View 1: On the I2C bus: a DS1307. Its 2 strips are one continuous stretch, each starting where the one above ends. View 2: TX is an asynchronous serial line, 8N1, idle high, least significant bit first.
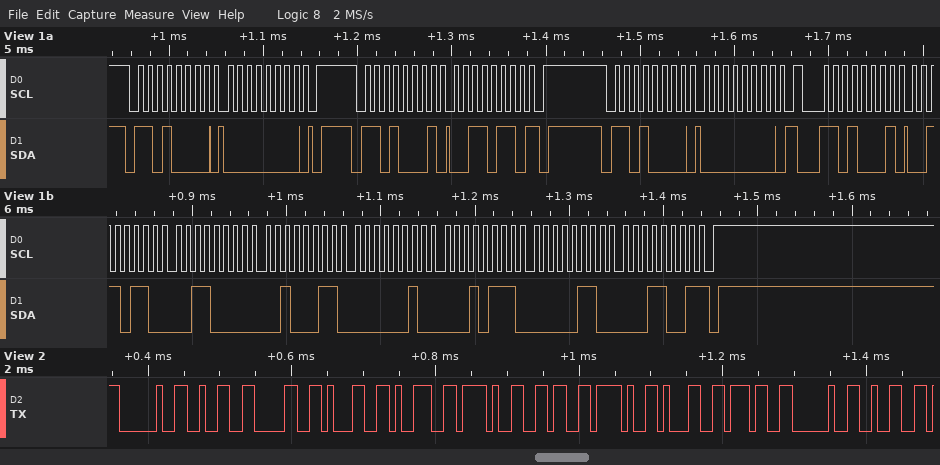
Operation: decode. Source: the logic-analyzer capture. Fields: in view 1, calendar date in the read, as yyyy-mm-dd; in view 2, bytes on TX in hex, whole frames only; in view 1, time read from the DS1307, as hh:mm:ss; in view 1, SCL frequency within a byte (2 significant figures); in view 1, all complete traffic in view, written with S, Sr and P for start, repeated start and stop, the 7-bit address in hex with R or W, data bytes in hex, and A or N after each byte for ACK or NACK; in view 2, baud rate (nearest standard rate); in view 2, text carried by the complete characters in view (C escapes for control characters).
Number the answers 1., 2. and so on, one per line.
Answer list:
1. 2019-06-17
2. 20 32 30 31 39 2F 36 2F 31 37 20 32
3. 23:30:36
4. 100 kHz
5. S 68W A 00 A P S 68R A 36 N P S 68W A 00 A Sr 68R A 36 A 30 A 23 A 02 A 17 A 06 A 19 N P
6. 115200 baud
7. " 2019/6/17 2"
